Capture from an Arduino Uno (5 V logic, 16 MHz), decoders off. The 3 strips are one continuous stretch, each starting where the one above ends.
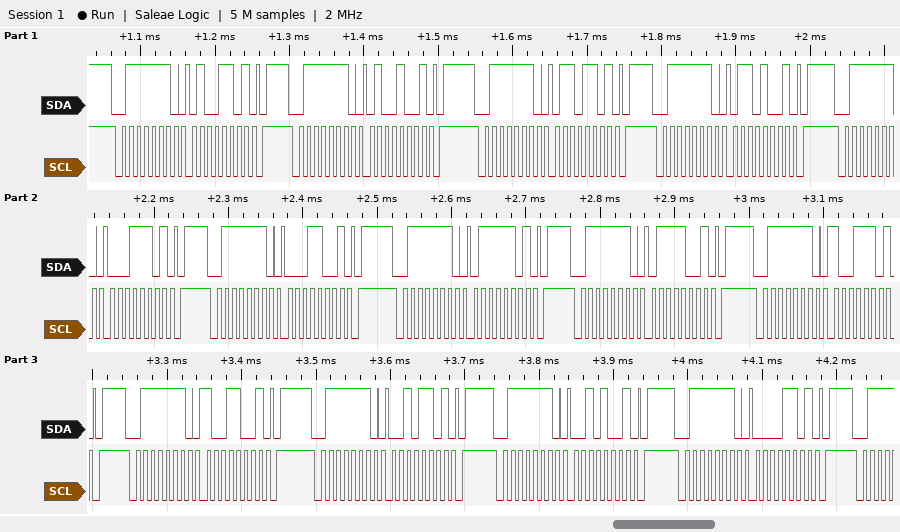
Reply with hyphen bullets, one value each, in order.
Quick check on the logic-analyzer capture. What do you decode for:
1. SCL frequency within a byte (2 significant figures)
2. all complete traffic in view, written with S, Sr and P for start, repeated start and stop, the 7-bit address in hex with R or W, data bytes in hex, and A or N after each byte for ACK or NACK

- 100 kHz
- S 3FW A 4D A P S 3FW A 49 A P S 3FW A 6D A P S 3FW A 69 A P S 3FW A 1D A P S 3FW A 19 A P S 3FW A 7D A P S 3FW A 79 A P S 3FW A 9D A P S 3FW A 99 A P S 3FW A 2D A P S 3FW A 29 A P S 3FW A 0D A P
